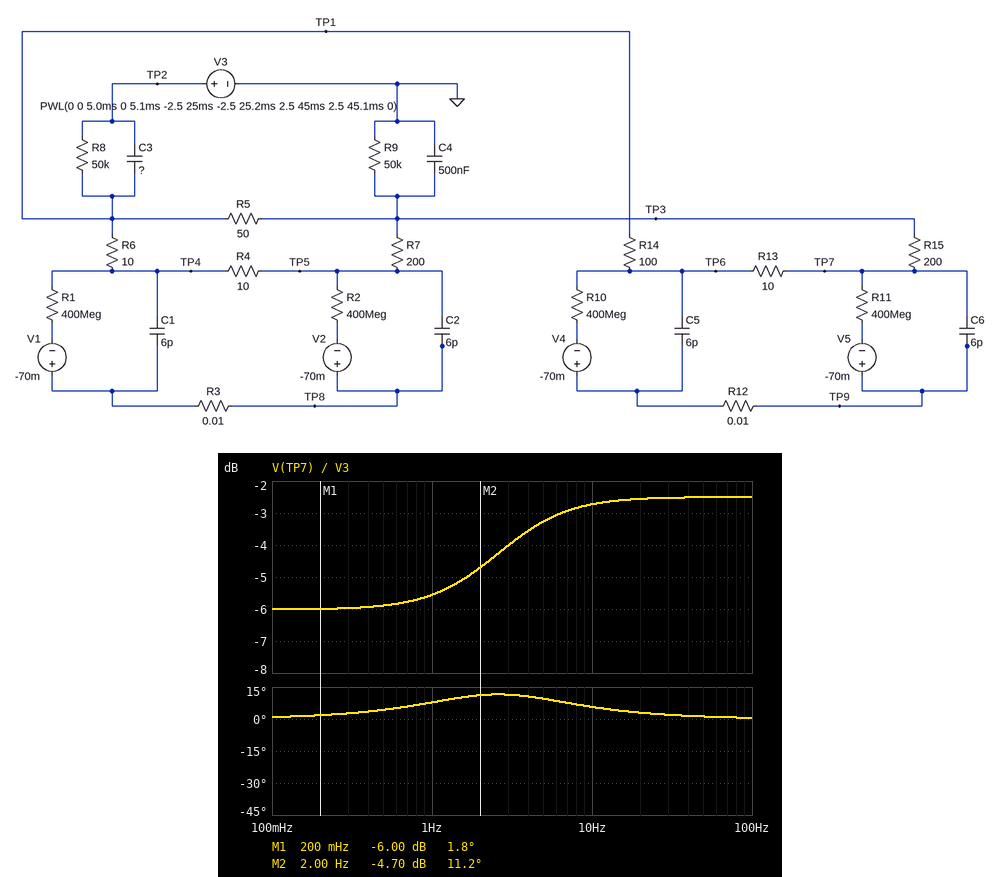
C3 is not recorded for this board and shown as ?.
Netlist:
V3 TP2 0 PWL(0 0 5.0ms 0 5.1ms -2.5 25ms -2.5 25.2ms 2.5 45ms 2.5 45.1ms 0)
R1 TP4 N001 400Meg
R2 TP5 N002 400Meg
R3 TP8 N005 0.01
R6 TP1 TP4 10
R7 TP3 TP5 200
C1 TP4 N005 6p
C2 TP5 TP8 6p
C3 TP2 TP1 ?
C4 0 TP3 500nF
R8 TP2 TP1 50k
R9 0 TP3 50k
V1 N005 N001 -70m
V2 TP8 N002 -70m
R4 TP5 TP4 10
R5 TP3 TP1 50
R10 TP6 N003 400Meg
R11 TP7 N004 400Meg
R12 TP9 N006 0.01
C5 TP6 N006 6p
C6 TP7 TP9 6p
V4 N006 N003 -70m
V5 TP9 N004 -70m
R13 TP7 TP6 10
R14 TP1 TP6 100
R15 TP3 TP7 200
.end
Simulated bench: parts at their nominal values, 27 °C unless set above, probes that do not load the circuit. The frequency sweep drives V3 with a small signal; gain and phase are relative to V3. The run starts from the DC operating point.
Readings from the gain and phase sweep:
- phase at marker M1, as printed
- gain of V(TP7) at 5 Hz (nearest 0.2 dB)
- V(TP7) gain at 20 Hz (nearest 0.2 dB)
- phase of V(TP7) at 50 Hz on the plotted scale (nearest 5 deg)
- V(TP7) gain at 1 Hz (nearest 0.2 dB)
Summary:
1.8 deg
-3.2 dB
-2.6 dB
0 deg
-5.6 dB
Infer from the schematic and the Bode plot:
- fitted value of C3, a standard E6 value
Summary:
1.5 µF
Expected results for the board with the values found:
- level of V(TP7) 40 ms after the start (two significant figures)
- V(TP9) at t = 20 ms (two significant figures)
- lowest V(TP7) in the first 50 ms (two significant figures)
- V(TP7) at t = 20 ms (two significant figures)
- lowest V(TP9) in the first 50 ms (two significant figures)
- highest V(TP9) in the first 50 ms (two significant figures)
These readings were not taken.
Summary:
1.9 V
-1.8 V
-1.9 V
-1.7 V
-1.9 V
2.0 V
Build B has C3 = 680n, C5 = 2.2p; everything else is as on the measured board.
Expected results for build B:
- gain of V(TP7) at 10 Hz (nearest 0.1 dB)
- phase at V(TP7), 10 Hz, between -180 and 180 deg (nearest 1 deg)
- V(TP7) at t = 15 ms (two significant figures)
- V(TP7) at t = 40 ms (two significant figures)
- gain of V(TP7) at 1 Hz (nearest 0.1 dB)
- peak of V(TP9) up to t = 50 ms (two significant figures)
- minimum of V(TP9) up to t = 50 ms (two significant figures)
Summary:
-5.0 dB
3 deg
-1.4 V
1.4 V
-6.0 dB
1.5 V
-1.5 V
